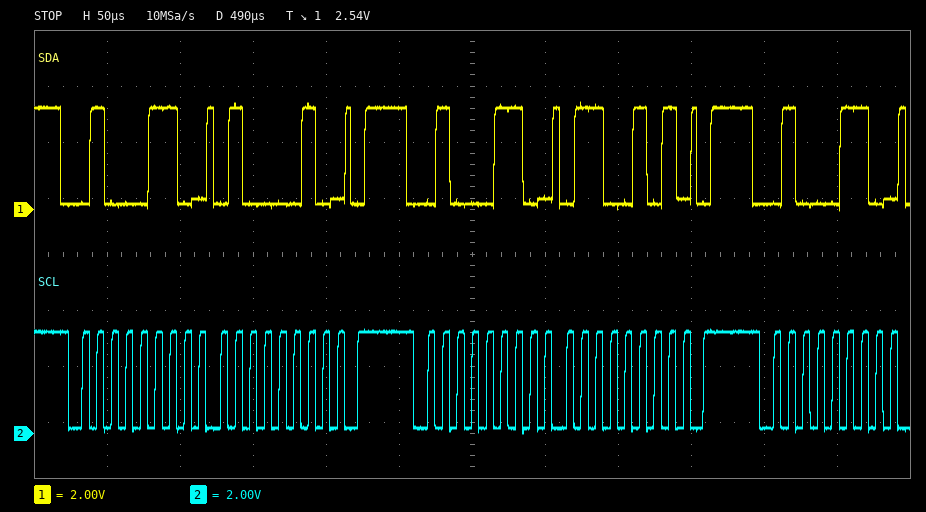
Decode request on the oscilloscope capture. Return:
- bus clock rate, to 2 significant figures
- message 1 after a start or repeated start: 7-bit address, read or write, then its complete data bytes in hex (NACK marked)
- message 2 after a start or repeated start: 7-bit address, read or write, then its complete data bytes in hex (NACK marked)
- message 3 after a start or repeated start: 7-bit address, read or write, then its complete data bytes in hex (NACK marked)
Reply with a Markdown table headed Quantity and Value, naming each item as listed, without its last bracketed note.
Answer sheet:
| Quantity | Value |
|---|---|
| bus clock rate, to 2 significant figures | 100 kHz |
| message 1 after a start or repeated start: 7-bit address, read or write, then its complete data bytes in hex | 0x23 write: 42 |
| message 2 after a start or repeated start: 7-bit address, read or write, then its complete data bytes in hex | 0x23 write: 65 |
| message 3 after a start or repeated start: 7-bit address, read or write, then its complete data bytes in hex | 0x23 write |
